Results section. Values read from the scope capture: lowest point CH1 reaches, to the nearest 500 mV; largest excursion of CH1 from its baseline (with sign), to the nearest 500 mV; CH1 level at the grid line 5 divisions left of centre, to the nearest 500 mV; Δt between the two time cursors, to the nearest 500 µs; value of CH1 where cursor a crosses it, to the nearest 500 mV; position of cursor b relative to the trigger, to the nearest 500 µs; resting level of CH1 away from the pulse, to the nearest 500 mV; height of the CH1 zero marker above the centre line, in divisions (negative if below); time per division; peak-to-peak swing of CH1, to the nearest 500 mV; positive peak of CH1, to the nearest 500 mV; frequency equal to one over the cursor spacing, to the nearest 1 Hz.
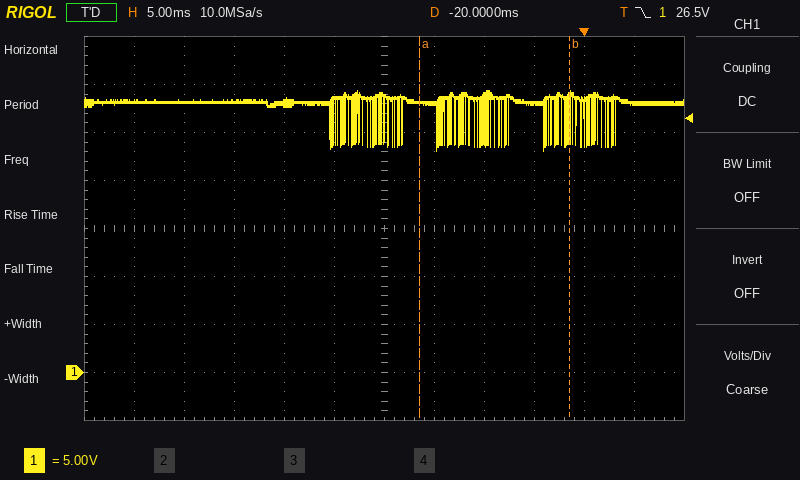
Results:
23.0 V
-5.0 V
28.0 V
15.0 ms
28.0 V
-1.5 ms
28.0 V
-3.0 div
5 ms
6.5 V
29.5 V
67 Hz
